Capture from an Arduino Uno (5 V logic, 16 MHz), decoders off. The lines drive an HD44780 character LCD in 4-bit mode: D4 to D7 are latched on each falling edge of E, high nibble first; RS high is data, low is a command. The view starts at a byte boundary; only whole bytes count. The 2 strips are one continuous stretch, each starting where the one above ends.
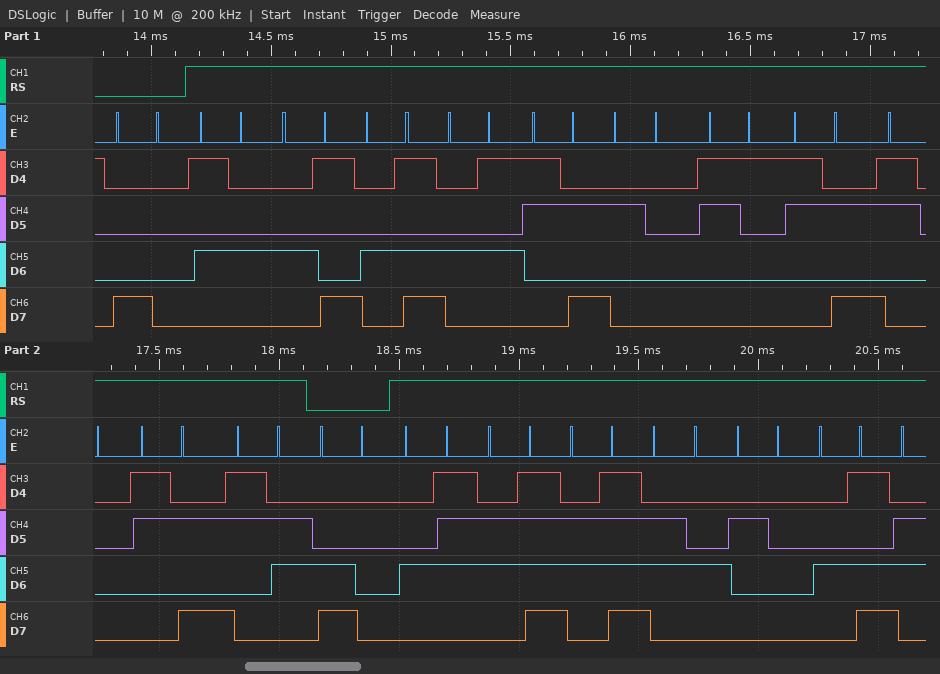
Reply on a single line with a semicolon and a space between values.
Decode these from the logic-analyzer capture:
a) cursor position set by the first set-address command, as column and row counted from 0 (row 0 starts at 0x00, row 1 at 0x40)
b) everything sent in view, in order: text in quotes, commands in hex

column 0, row 0; 0x80 "TIME: 1:0:6" 0xC0 "Good M"
